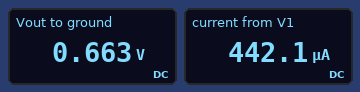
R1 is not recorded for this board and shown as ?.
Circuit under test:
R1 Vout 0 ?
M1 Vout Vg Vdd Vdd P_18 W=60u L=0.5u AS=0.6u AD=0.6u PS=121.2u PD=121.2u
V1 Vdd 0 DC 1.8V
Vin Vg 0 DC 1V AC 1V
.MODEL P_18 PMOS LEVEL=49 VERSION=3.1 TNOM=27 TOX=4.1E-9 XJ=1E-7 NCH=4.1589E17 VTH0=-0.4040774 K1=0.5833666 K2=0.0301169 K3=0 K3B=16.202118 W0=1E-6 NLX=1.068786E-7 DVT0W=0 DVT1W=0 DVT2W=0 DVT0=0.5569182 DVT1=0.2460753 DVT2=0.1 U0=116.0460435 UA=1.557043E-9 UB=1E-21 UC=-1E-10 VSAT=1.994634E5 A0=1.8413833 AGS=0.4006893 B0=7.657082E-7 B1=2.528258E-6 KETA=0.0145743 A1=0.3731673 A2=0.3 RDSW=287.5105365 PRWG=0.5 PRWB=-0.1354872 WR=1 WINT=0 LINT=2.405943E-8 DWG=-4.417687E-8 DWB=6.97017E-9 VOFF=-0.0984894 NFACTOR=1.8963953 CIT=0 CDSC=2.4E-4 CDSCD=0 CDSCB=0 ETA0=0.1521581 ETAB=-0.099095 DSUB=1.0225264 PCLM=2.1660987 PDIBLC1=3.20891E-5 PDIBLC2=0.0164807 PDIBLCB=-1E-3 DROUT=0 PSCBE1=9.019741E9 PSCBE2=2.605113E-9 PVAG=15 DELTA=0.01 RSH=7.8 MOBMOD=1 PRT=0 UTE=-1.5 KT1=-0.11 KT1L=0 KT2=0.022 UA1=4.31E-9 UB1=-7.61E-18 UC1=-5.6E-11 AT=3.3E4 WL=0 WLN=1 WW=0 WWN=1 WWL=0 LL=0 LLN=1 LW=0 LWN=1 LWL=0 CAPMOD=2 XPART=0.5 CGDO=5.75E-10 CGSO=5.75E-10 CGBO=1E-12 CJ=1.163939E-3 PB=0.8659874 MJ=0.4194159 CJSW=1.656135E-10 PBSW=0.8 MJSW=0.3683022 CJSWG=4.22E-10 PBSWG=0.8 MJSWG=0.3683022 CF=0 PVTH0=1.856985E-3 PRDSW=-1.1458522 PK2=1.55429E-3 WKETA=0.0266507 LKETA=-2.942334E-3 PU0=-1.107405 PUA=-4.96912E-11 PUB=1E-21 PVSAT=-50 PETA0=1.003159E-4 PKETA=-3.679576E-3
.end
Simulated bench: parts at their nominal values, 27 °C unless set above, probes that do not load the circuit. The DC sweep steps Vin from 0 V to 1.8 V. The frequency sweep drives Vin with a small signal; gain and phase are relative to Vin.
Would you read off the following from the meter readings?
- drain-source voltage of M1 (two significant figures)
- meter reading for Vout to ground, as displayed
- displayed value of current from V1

-1.1 V
0.663 V
442.1 µA
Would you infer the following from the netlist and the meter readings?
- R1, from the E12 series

1.5 kΩ
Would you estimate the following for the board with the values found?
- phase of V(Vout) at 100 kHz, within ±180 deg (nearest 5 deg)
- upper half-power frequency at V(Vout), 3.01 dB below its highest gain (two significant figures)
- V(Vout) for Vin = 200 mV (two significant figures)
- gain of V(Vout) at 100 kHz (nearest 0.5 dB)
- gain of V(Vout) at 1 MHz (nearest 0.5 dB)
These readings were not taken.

155 deg
220 kHz
1.6 V
9.5 dB
-3.0 dB
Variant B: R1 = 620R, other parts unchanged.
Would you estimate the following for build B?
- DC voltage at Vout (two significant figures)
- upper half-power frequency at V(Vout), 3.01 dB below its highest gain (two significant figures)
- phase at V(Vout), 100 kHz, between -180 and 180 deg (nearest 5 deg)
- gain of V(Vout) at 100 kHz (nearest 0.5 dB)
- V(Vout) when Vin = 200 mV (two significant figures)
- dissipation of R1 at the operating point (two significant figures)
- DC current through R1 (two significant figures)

280 mV
560 kHz
170 deg
3.0 dB
1.4 V
130 µW
450 µA
